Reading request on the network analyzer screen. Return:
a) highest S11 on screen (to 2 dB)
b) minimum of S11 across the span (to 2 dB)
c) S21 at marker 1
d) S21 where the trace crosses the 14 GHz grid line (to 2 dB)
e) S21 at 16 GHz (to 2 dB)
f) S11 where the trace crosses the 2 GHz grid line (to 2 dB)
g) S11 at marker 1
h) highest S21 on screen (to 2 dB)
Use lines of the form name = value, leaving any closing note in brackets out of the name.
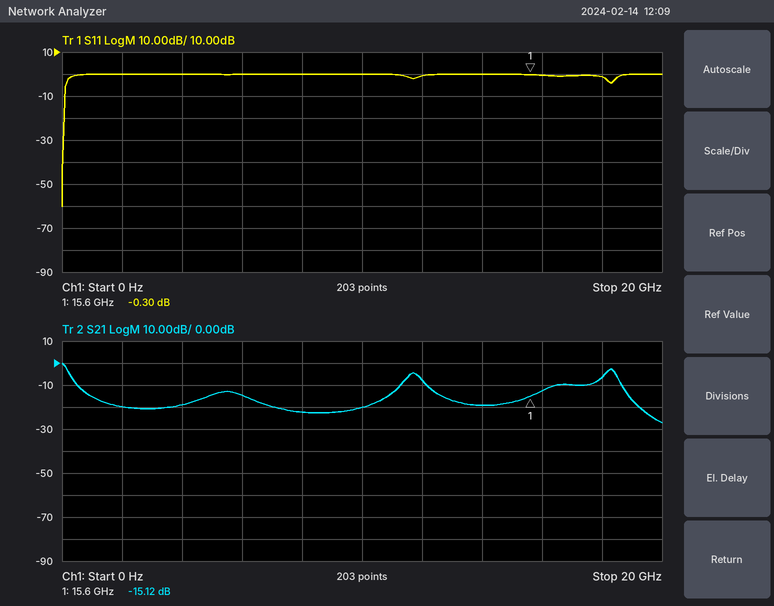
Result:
highest S11 on screen = 0 dB
minimum of S11 across the span = -60 dB
S21 at marker 1 = -15.12 dB
S21 where the trace crosses the 14 GHz grid line = -20 dB
S21 at 16 GHz = -12 dB
S11 where the trace crosses the 2 GHz grid line = 0 dB
S11 at marker 1 = -0.30 dB
highest S21 on screen = 0 dB
